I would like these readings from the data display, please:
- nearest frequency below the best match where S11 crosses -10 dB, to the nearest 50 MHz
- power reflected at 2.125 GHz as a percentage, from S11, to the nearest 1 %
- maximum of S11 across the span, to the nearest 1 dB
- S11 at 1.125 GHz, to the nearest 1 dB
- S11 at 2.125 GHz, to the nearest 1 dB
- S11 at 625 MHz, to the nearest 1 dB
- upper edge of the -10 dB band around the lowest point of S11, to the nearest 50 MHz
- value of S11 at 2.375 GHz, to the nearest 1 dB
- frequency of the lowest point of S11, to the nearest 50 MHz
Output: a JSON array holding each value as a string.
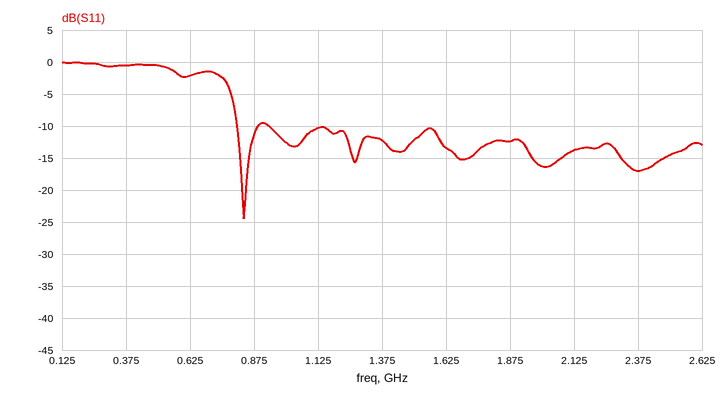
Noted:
["800 MHz", "4 %", "0 dB", "-10 dB", "-14 dB", "-2 dB", "900 MHz", "-17 dB", "850 MHz"]
